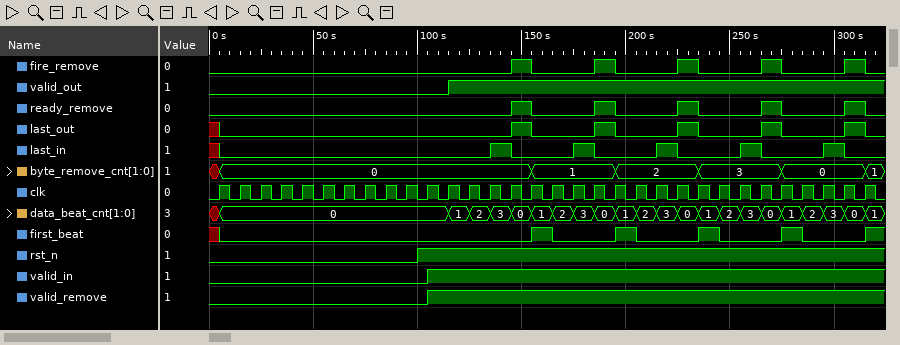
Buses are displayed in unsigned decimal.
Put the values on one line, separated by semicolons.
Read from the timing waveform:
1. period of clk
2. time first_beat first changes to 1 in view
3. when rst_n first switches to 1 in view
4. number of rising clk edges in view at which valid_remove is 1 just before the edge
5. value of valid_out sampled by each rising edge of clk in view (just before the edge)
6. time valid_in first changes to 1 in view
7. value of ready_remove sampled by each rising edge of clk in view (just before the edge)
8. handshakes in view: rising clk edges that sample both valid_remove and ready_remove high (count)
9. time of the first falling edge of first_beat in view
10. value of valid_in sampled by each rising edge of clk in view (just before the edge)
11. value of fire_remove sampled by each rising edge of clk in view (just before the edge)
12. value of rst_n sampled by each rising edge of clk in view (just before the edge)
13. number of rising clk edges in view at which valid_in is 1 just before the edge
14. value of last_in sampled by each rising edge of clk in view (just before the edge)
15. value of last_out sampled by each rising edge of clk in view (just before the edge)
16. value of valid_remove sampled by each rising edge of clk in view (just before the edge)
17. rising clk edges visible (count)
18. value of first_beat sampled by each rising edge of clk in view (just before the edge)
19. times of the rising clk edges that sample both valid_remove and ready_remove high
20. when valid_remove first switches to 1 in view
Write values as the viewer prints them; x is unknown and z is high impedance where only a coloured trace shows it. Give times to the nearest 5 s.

10 s; 155 s; 100 s; 21; 0 0 0 0 0 0 0 0 0 0 0 0 1 1 1 1 1 1 1 1 1 1 1 1 1 1 1 1 1 1 1 1; 105 s; 0 0 0 0 0 0 0 0 0 0 0 0 0 0 0 1 0 0 0 1 0 0 0 1 0 0 0 1 0 0 0 1; 5; 165 s; 0 0 0 0 0 0 0 0 0 0 0 1 1 1 1 1 1 1 1 1 1 1 1 1 1 1 1 1 1 1 1 1; 0 0 0 0 0 0 0 0 0 0 0 0 0 0 0 1 0 0 0 1 0 0 0 1 0 0 0 1 0 0 0 1; 0 0 0 0 0 0 0 0 0 0 1 1 1 1 1 1 1 1 1 1 1 1 1 1 1 1 1 1 1 1 1 1; 21; x 0 0 0 0 0 0 0 0 0 0 0 0 0 1 0 0 0 1 0 0 0 1 0 0 0 1 0 0 0 1 0; x 0 0 0 0 0 0 0 0 0 0 0 0 0 0 1 0 0 0 1 0 0 0 1 0 0 0 1 0 0 0 1; 0 0 0 0 0 0 0 0 0 0 0 1 1 1 1 1 1 1 1 1 1 1 1 1 1 1 1 1 1 1 1 1; 32; x 0 0 0 0 0 0 0 0 0 0 0 0 0 0 0 1 0 0 0 1 0 0 0 1 0 0 0 1 0 0 0; 155 s, 195 s, 235 s, 275 s, 315 s; 105 s
